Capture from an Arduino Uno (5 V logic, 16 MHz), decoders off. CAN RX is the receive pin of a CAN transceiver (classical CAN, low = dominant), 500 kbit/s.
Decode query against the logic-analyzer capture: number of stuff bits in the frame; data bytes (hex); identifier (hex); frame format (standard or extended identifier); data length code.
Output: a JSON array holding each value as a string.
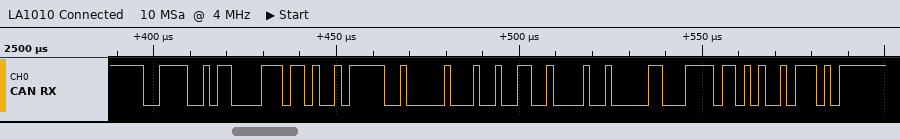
["3", "69 7D 00 93 21 20 8F", "0x3CB", "standard", "7"]
